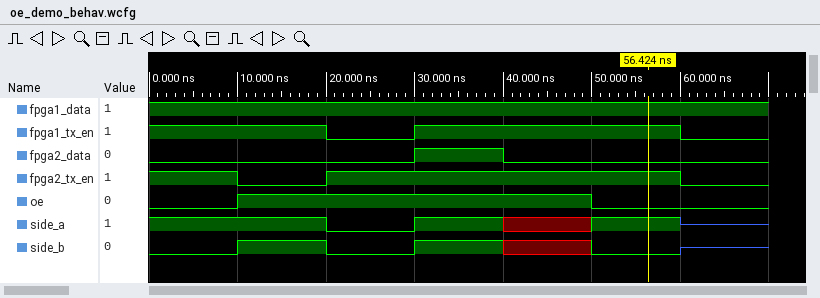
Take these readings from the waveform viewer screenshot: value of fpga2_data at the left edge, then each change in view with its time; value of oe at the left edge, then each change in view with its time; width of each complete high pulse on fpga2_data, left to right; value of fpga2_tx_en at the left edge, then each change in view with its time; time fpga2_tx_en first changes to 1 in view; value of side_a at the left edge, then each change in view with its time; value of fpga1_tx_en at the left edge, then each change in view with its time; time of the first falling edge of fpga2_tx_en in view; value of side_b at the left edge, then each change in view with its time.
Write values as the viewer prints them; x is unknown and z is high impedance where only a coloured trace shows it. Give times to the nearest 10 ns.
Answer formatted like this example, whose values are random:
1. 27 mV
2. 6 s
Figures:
1. 0, 1 at 30 ns, 0 at 40 ns
2. 0, 1 at 10 ns, 0 at 50 ns
3. 10 ns
4. 1, 0 at 10 ns, 1 at 20 ns, 0 at 60 ns
5. 20 ns
6. 1, 0 at 20 ns, 1 at 30 ns, x at 40 ns, 1 at 50 ns, z at 60 ns
7. 1, 0 at 20 ns, 1 at 30 ns, 0 at 60 ns
8. 10 ns
9. 0, 1 at 10 ns, 0 at 20 ns, 1 at 30 ns, x at 40 ns, 0 at 50 ns, z at 60 ns
